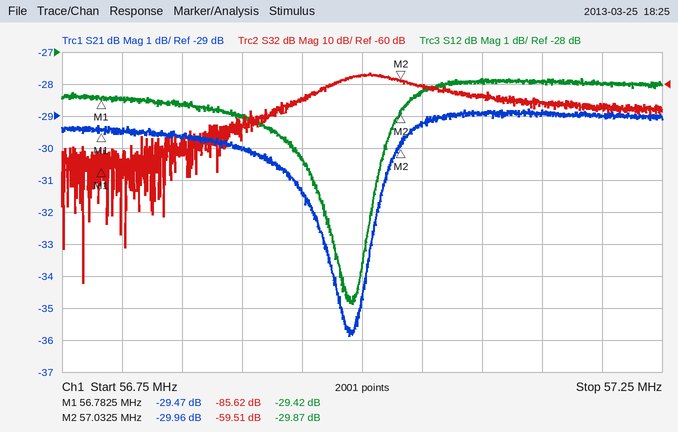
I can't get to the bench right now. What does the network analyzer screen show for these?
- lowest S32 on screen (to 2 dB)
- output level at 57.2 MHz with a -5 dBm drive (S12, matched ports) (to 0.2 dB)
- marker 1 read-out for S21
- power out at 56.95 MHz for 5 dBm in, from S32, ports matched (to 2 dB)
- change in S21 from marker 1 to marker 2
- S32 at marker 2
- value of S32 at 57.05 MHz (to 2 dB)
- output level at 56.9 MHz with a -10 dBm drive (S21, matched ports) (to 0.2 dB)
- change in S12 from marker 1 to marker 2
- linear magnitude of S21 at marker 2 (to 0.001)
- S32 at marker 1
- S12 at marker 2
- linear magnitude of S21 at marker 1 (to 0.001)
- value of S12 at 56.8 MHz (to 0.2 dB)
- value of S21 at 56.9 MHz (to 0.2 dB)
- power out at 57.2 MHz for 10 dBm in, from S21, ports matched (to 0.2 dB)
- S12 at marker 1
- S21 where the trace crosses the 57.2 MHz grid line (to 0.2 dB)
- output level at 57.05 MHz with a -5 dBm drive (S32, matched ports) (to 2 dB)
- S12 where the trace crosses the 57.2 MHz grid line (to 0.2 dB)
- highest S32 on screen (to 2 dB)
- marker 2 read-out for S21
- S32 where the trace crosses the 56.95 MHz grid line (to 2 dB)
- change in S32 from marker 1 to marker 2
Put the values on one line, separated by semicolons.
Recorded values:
-122 dB; -34.0 dBm; -29.47 dB; -60 dBm; -0.49 dB; -59.51 dB; -60 dB; -40.0 dBm; -0.45 dB; 0.032; -85.62 dB; -29.87 dB; 0.034; -29.4 dB; -30.0 dB; -19.0 dBm; -29.42 dB; -29.0 dB; -66 dBm; -29.0 dB; -56 dB; -29.96 dB; -64 dB; 26.11 dB
